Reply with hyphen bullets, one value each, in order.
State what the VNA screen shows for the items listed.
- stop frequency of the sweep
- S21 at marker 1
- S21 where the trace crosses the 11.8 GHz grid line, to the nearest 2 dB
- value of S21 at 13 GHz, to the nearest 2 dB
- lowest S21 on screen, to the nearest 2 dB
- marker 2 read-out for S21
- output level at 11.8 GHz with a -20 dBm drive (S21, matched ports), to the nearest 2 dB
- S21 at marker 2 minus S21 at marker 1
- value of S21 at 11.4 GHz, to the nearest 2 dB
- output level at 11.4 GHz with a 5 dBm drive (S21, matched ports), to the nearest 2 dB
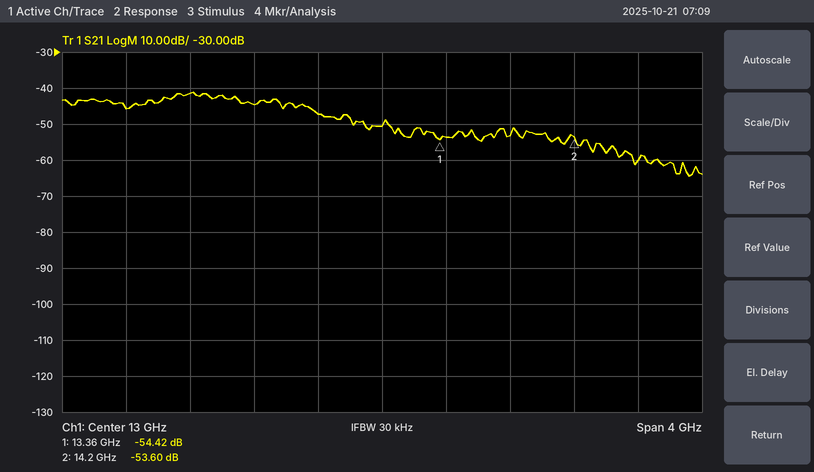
- 15 GHz
- -54.42 dB
- -42 dB
- -50 dB
- -64 dB
- -53.60 dB
- -62 dBm
- 0.82 dB
- -46 dB
- -40 dBm
